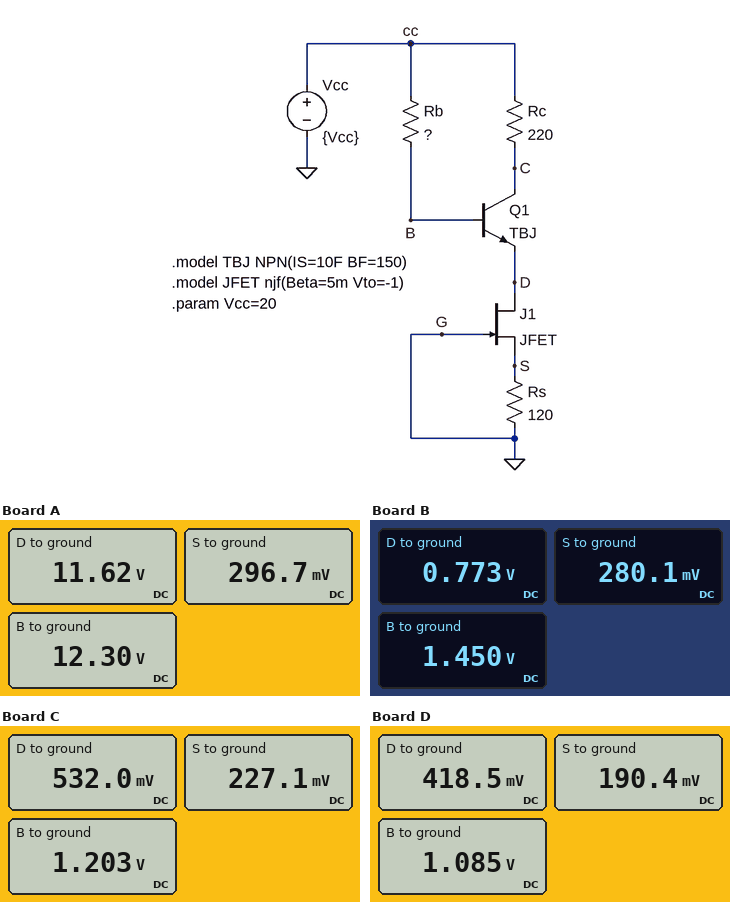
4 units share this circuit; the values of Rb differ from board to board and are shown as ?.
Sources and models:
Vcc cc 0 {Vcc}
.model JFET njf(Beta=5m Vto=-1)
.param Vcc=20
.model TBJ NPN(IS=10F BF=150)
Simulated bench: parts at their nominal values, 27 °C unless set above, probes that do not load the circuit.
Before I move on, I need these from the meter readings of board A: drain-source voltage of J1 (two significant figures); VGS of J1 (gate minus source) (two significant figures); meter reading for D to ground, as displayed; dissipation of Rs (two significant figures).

11 V
-300 mV
11.62 V
730 µW
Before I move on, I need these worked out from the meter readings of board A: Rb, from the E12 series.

470 kΩ
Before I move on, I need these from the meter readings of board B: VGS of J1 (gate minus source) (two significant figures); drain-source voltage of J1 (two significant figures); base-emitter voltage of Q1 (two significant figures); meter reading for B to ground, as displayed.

-280 mV
490 mV
680 mV
1.450 V
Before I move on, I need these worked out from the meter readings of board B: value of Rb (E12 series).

1.2 MΩ
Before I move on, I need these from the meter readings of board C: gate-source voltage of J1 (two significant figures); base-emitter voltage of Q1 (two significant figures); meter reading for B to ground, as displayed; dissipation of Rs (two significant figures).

-230 mV
670 mV
1.203 V
430 µW
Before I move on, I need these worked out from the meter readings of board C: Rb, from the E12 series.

1.5 MΩ
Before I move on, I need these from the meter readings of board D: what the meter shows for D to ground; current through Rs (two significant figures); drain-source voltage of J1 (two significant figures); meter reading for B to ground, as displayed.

418.5 mV
1.6 mA
230 mV
1.085 V
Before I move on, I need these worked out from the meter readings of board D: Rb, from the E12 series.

1.8 MΩ
